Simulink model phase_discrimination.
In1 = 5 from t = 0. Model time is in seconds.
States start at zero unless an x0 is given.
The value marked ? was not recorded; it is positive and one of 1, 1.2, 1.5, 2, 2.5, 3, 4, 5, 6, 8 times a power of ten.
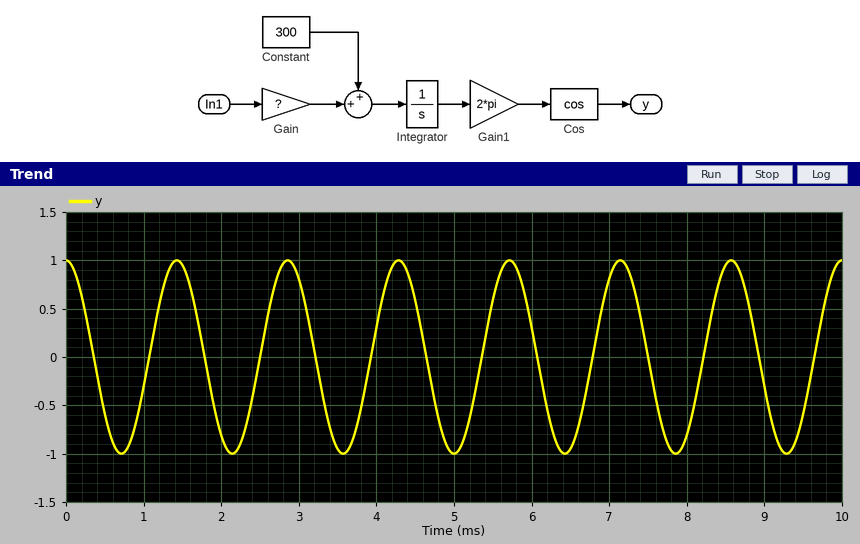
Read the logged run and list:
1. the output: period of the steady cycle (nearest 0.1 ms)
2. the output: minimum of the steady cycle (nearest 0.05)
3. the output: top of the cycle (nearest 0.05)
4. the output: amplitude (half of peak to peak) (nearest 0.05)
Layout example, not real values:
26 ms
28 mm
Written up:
1.4 ms
-1.00
1.00
1.00
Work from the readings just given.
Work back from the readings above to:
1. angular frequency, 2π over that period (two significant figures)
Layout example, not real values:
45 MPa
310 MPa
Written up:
4.5 rad/ms
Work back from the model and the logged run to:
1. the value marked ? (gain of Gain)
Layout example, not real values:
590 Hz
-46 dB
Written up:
80
